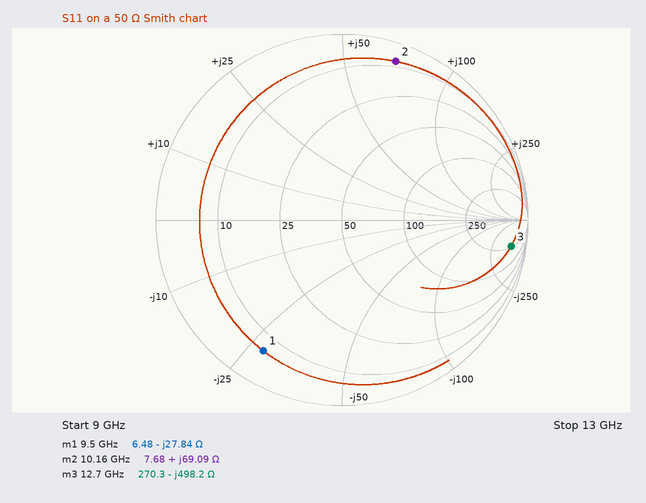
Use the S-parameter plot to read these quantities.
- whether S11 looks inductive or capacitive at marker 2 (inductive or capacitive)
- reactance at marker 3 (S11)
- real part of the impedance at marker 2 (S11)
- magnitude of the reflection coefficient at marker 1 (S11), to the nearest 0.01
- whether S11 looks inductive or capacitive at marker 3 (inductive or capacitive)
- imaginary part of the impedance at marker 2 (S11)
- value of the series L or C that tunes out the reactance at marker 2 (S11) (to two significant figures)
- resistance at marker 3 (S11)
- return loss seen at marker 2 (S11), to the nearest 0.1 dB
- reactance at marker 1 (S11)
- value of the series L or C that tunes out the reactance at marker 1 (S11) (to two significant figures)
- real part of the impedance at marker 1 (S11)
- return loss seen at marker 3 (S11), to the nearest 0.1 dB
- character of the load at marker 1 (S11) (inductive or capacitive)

inductive
-498.2 Ω
7.68 Ω
0.82
capacitive
+69.09 Ω
230 fF
270.3 Ω
0.9 dB
-27.84 Ω
470 pH
6.48 Ω
0.7 dB
capacitive
